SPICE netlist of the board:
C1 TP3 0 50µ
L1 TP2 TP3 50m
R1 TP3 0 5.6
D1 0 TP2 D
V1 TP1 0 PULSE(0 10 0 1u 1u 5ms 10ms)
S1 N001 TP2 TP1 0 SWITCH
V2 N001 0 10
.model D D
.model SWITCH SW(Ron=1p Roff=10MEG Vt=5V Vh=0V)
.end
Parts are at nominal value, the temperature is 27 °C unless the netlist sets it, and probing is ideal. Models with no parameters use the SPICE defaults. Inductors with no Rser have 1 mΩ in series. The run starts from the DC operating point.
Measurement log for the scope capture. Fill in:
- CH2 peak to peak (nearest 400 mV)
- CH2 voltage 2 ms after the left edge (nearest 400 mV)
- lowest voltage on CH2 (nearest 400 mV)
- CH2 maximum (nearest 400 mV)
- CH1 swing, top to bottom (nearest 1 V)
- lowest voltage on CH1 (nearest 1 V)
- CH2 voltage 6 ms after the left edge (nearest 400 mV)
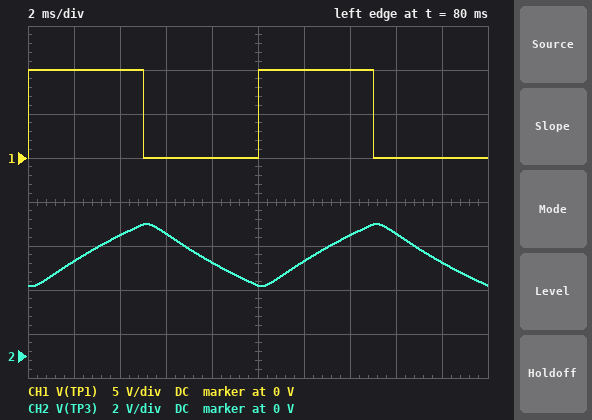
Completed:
2.8 V
4.4 V
3.2 V
6.0 V
10 V
0 V
5.6 V
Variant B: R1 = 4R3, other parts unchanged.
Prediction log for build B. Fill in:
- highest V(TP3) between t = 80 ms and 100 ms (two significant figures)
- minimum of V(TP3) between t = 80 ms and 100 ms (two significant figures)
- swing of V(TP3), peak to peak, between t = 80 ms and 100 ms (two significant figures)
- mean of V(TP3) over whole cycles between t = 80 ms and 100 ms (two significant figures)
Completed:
5.7 V
3.5 V
2.2 V
4.6 V
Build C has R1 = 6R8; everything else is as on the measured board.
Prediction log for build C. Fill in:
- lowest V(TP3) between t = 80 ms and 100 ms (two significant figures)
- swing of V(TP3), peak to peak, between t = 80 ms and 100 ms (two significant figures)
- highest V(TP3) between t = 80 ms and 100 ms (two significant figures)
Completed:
2.9 V
3.4 V
6.3 V
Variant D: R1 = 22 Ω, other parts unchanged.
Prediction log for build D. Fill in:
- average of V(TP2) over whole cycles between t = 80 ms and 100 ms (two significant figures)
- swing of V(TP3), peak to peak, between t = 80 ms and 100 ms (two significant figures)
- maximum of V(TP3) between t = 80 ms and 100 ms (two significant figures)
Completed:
5.0 V
9.3 V
9.7 V
